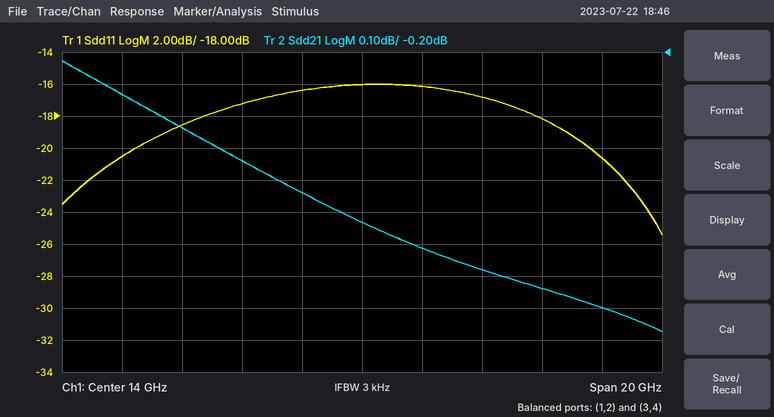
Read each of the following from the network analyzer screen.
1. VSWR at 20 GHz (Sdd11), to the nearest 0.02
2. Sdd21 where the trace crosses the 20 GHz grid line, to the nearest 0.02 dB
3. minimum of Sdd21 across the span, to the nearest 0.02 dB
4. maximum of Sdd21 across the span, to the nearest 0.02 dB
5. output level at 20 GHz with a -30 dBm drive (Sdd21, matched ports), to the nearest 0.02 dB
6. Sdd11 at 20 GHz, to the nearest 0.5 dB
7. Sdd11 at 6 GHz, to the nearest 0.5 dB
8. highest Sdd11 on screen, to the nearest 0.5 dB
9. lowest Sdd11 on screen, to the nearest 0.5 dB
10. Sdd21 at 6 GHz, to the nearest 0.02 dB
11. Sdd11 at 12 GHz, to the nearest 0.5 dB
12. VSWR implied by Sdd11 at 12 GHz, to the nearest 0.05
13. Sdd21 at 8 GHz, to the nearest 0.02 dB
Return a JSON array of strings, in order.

["1.28", "-0.94 dB", "-1.08 dB", "-0.22 dB", "-30.94 dBm", "-18.0 dB", "-20.5 dB", "-16.0 dB", "-25.5 dB", "-0.34 dB", "-16.5 dB", "1.35", "-0.44 dB"]
